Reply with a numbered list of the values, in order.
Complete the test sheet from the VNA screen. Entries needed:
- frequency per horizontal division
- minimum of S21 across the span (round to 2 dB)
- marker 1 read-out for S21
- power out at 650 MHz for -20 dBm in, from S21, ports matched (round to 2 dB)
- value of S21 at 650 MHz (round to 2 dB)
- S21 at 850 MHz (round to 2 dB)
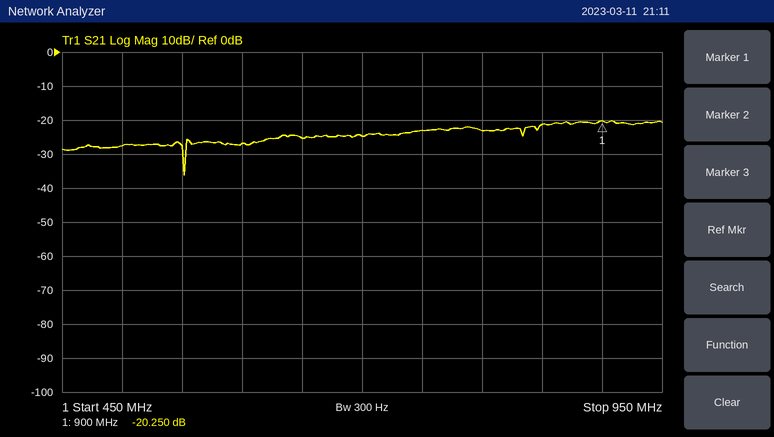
1. 50 MHz
2. -36 dB
3. -20.250 dB
4. -46 dBm
5. -26 dB
6. -22 dB
